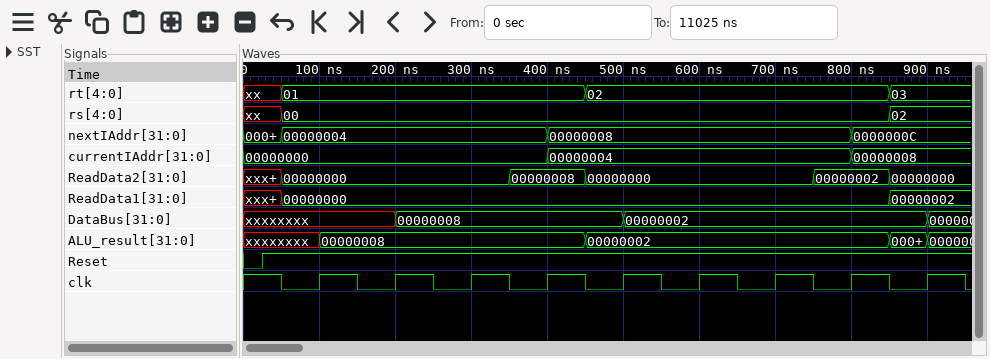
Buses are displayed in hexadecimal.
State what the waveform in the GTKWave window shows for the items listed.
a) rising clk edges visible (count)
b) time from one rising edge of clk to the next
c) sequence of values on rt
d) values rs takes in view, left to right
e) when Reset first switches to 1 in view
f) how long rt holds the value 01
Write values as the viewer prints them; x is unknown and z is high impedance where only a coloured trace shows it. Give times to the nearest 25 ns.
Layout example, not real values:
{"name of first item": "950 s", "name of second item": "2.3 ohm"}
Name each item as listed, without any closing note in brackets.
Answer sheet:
{"rising clk edges visible": "9", "time from one rising edge of clk to the next": "100 ns", "sequence of values on rt": "xx, 01, 02, 03", "values rs takes in view, left to right": "xx, 00, 02", "when Reset first switches to 1 in view": "25 ns", "how long rt holds the value 01": "400 ns"}
